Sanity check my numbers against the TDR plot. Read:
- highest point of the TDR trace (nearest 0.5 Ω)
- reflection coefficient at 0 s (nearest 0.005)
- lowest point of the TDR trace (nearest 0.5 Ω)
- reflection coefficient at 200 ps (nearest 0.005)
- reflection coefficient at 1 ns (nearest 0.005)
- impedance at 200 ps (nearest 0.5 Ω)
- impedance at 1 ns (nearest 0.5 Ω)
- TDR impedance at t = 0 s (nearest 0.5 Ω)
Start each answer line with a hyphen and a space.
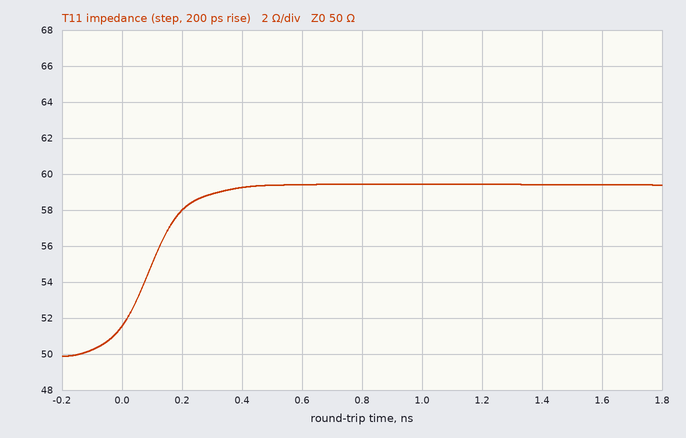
- 59.5 Ω
- +0.015
- 50.0 Ω
- +0.075
- +0.085
- 58.0 Ω
- 59.5 Ω
- 51.5 Ω
